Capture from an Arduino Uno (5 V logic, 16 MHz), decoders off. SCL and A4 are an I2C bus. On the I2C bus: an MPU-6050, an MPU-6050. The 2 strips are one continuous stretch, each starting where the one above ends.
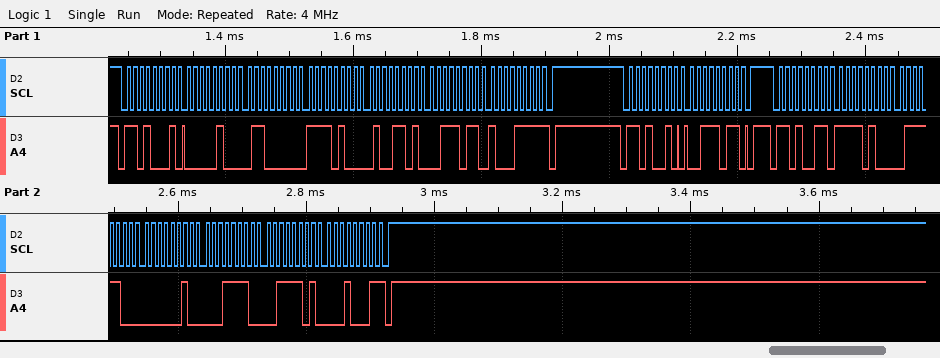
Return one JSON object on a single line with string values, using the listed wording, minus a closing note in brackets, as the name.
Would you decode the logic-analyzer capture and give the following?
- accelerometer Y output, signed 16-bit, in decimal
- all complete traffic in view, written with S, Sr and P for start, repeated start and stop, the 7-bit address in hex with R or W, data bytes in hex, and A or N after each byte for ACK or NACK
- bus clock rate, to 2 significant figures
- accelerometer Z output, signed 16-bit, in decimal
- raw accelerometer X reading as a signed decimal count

{"accelerometer Y output, signed 16-bit, in decimal": "542", "all complete traffic in view, written with S, Sr and P for start, repeated start and stop, the 7-bit address in hex with R or W, data bytes in hex, and A or N after each byte for ACK or NACK": "S 68R A 04 A 60 A F4 A 4D A 3B A 8F N P S 69W A 3B A P S 69R A F4 A 7C A 02 A 1E A 3D A 11 N P", "bus clock rate, to 2 significant figures": "100 kHz", "accelerometer Z output, signed 16-bit, in decimal": "15633", "raw accelerometer X reading as a signed decimal count": "-2948"}
